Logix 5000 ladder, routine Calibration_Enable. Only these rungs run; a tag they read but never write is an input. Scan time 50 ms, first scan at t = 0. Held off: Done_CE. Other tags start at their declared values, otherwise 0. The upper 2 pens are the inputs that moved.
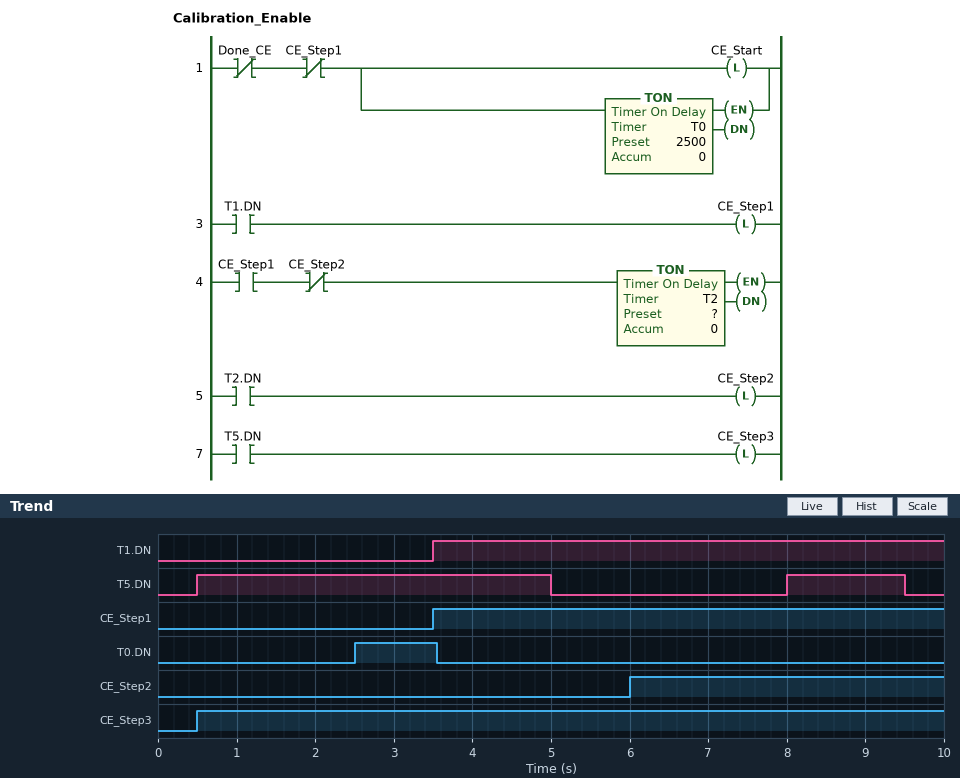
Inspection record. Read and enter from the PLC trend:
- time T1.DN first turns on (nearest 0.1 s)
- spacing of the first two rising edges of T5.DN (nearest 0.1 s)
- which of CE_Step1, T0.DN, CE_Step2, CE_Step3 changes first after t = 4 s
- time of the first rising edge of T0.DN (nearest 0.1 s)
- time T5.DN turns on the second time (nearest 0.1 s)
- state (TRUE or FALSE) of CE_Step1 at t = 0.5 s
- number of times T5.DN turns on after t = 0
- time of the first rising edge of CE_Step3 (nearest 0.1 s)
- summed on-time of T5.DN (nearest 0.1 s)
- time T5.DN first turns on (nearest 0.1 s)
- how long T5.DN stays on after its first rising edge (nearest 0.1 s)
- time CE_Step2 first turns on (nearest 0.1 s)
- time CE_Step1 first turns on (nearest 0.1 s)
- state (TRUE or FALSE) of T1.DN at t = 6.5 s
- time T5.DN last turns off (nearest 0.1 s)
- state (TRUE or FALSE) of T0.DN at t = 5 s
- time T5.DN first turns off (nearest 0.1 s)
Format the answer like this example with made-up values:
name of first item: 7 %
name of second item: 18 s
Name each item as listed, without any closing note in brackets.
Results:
time T1.DN first turns on: 3.5 s
spacing of the first two rising edges of T5.DN: 7.5 s
which of CE_Step1, T0.DN, CE_Step2, CE_Step3 changes first after t = 4 s: CE_Step2
time of the first rising edge of T0.DN: 2.5 s
time T5.DN turns on the second time: 8.0 s
state (TRUE or FALSE) of CE_Step1 at t = 0.5 s: FALSE
number of times T5.DN turns on after t = 0: 2
time of the first rising edge of CE_Step3: 0.5 s
summed on-time of T5.DN: 6.0 s
time T5.DN first turns on: 0.5 s
how long T5.DN stays on after its first rising edge: 4.5 s
time CE_Step2 first turns on: 6.0 s
time CE_Step1 first turns on: 3.5 s
state (TRUE or FALSE) of T1.DN at t = 6.5 s: TRUE
time T5.DN last turns off: 9.5 s
state (TRUE or FALSE) of T0.DN at t = 5 s: FALSE
time T5.DN first turns off: 5.0 s
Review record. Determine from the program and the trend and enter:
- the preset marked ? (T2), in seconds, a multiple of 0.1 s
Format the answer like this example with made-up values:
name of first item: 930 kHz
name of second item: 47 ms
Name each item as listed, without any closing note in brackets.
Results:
the preset marked ? (T2), in seconds, a multiple of 0.1 s: 2.5 s
